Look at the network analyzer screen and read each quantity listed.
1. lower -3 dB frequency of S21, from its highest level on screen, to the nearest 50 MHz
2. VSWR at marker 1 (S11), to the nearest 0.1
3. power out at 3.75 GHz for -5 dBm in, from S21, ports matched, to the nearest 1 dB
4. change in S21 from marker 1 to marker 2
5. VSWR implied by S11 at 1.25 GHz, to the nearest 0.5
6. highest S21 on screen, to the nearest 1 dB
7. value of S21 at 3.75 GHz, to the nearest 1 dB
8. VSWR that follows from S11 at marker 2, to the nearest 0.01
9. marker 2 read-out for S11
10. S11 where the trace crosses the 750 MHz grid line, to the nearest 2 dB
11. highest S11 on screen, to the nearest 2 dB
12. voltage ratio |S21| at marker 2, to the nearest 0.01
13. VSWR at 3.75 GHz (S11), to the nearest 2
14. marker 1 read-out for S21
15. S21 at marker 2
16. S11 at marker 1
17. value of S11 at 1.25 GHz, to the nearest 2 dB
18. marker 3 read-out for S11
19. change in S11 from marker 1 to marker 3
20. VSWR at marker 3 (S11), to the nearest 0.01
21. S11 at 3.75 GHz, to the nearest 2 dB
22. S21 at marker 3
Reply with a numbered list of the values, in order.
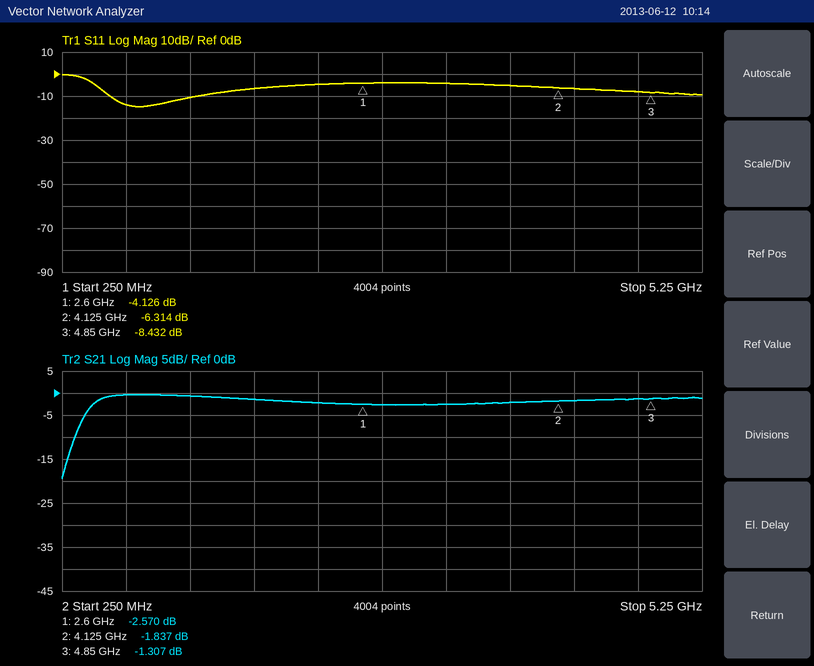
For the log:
1. 450 MHz
2. 4.3
3. -7 dBm
4. 0.733 dB
5. 2.0
6. 0 dB
7. -2 dB
8. 2.87
9. -6.314 dB
10. -14 dB
11. 0 dB
12. 0.81
13. 4
14. -2.570 dB
15. -1.837 dB
16. -4.126 dB
17. -10 dB
18. -8.432 dB
19. -4.306 dB
20. 2.22
21. -6 dB
22. -1.307 dB
